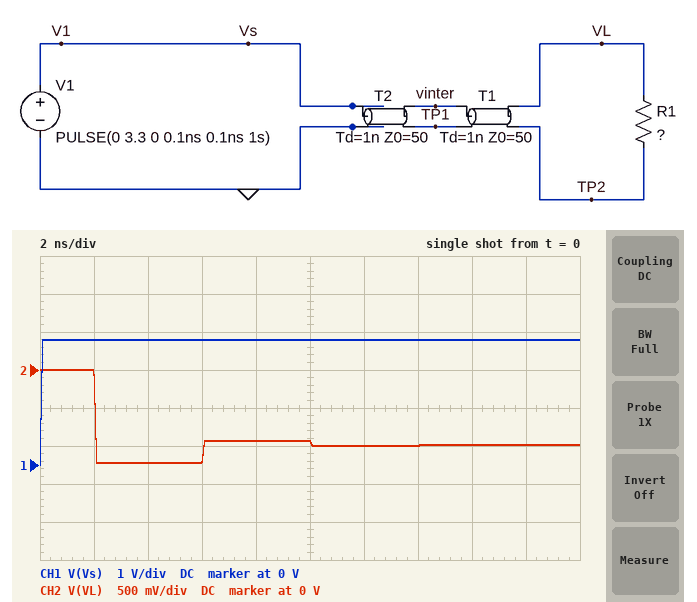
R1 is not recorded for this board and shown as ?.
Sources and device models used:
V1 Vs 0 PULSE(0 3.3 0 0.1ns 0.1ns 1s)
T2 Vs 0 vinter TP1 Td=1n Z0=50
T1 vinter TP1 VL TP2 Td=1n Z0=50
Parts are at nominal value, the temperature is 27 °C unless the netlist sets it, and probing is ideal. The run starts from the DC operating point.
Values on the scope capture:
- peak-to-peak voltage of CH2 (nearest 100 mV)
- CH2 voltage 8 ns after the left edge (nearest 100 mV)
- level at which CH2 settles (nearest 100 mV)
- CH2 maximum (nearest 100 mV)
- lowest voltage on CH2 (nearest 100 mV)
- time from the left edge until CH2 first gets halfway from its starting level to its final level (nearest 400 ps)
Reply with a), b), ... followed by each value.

a) 1.2 V
b) -900 mV
c) -1.0 V
d) 0 V
e) -1.2 V
f) 2.0 ns
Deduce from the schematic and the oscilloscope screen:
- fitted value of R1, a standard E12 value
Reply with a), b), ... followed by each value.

a) 82 Ω
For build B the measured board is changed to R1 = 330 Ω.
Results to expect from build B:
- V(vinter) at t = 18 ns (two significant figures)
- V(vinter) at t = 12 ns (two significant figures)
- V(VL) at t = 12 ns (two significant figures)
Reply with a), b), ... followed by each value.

a) -660 mV
b) -350 mV
c) -340 mV
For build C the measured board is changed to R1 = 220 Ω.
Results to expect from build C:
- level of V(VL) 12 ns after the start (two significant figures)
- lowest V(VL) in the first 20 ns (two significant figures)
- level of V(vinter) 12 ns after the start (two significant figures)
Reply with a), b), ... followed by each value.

a) -460 mV
b) -600 mV
c) -470 mV
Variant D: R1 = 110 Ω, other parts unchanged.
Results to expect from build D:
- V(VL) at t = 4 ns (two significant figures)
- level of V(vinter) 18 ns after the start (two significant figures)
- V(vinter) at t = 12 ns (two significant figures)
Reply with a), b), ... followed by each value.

a) -1.0 V
b) -770 mV
c) -790 mV
